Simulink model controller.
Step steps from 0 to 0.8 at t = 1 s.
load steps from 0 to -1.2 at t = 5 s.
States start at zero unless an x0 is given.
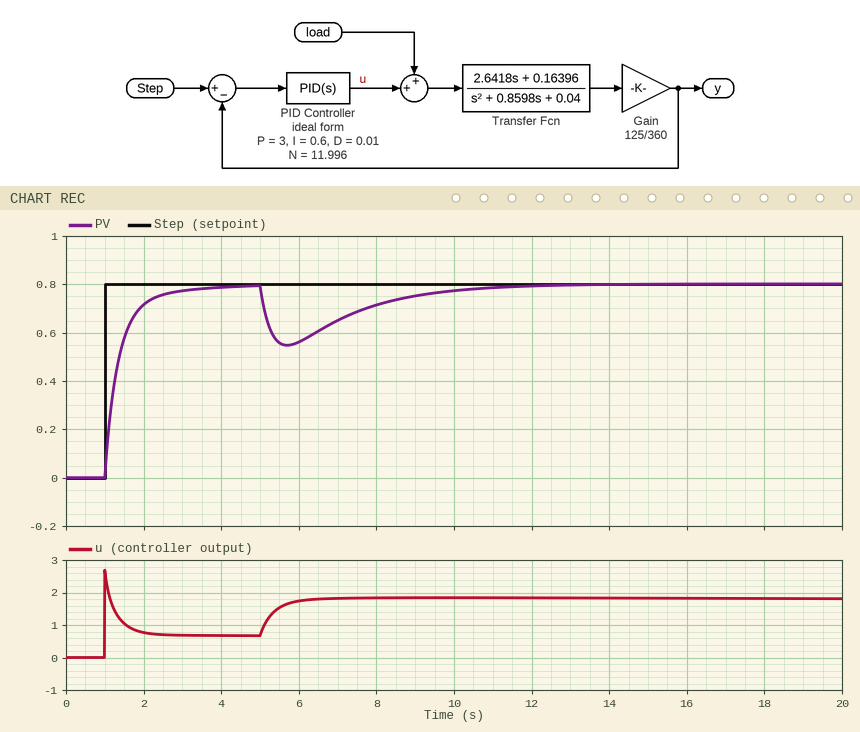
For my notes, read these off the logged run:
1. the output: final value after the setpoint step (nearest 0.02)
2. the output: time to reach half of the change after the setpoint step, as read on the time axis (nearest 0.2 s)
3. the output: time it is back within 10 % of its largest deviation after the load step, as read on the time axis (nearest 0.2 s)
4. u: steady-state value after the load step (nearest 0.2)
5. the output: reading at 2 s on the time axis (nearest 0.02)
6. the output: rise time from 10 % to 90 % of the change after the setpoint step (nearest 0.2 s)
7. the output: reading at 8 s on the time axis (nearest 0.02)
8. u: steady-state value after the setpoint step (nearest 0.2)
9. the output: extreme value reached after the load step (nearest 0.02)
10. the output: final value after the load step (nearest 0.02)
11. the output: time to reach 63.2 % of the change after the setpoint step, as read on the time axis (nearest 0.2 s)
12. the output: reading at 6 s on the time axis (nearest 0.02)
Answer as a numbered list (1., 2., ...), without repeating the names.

1. 0.80
2. 1.2 s
3. 10.2 s
4. 1.8
5. 0.72
6. 1.0 s
7. 0.72
8. 0.6
9. 0.54
10. 0.80
11. 1.4 s
12. 0.56
